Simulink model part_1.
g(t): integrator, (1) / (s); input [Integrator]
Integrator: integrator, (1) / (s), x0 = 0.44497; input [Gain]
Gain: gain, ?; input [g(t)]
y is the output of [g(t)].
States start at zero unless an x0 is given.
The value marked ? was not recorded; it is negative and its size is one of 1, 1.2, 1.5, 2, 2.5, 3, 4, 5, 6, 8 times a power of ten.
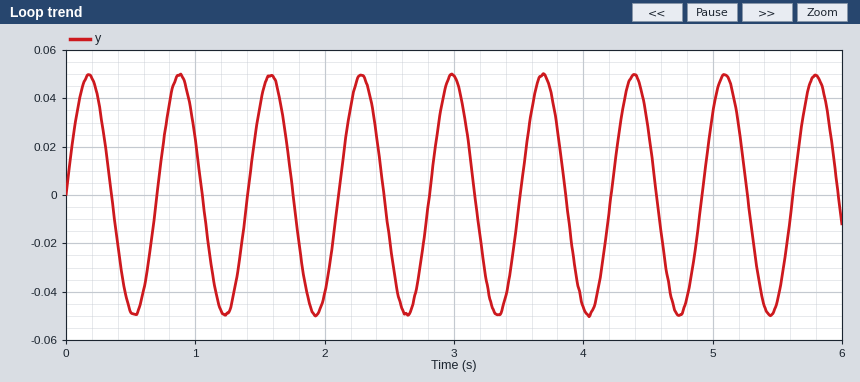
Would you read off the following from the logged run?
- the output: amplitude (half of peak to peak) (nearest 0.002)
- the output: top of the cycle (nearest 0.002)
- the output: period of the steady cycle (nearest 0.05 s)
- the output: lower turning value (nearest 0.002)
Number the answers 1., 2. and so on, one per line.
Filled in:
1. 0.050
2. 0.050
3. 0.70 s
4. -0.050
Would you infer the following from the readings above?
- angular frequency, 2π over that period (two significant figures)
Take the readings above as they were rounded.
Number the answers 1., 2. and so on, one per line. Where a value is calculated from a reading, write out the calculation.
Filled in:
1. 2π / 0.7 = 9.0 rad/s
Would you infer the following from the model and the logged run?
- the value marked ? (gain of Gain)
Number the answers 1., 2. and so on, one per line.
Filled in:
1. -80
